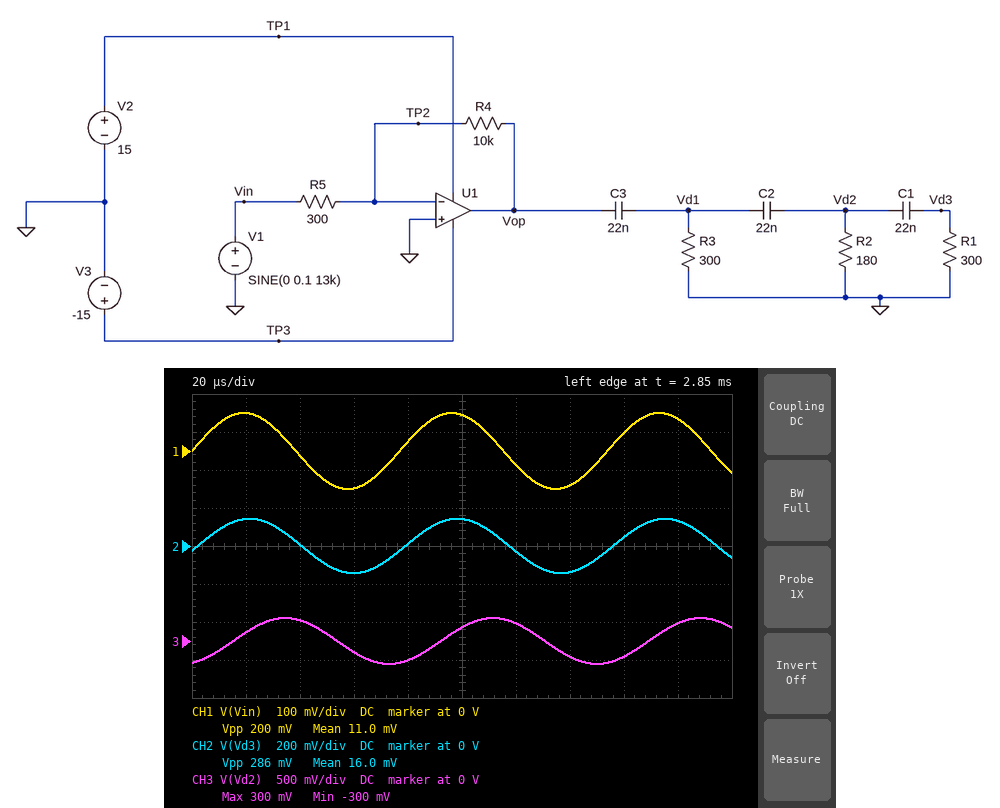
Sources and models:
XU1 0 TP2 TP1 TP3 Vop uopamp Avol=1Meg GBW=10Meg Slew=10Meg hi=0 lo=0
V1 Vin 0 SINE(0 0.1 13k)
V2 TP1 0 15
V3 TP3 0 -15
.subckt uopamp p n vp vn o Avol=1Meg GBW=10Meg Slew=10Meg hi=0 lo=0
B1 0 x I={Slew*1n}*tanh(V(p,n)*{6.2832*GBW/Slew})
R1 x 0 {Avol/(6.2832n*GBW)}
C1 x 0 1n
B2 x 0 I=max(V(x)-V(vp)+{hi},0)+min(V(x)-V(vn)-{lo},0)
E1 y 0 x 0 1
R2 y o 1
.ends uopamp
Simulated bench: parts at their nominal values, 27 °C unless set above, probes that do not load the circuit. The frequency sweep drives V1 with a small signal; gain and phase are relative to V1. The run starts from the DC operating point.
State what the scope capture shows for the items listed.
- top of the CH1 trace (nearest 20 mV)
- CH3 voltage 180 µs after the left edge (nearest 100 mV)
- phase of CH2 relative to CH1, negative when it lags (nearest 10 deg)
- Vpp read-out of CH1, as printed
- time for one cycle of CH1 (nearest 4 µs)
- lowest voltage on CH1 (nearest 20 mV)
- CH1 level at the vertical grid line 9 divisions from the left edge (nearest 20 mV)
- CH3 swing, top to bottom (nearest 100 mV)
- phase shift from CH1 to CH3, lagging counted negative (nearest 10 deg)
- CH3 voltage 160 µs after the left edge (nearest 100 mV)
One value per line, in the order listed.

100 mV
200 mV
-10 deg
200 mV
76 µs
-100 mV
80 mV
600 mV
-70 deg
-200 mV
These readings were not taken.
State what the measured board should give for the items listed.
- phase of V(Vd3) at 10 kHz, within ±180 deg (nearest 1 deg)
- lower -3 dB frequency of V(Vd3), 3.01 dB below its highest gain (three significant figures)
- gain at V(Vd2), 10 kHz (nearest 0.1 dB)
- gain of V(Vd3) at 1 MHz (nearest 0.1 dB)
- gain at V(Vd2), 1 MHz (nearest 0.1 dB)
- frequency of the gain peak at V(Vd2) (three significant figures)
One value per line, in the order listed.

6 deg
85.9 kHz
6.7 dB
19.2 dB
19.2 dB
207 kHz
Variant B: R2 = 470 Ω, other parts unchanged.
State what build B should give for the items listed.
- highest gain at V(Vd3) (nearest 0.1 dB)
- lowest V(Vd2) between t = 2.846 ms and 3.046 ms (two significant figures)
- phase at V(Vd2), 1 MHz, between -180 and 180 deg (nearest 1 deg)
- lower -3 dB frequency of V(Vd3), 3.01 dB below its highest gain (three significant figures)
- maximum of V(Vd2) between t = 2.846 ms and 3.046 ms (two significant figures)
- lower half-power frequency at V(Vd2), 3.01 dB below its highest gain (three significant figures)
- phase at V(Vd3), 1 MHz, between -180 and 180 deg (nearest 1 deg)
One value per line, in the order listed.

27.7 dB
-510 mV
112 deg
69.0 kHz
510 mV
63.8 kHz
113 deg
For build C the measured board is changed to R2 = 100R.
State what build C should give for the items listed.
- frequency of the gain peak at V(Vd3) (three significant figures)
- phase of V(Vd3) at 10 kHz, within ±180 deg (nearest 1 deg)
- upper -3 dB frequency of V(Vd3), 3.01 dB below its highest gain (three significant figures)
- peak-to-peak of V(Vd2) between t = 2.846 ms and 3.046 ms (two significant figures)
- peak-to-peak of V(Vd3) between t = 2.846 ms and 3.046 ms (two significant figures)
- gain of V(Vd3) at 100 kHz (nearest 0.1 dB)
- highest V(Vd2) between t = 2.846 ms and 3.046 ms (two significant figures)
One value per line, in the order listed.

248 kHz
14 deg
599 kHz
380 mV
180 mV
22.4 dB
190 mV
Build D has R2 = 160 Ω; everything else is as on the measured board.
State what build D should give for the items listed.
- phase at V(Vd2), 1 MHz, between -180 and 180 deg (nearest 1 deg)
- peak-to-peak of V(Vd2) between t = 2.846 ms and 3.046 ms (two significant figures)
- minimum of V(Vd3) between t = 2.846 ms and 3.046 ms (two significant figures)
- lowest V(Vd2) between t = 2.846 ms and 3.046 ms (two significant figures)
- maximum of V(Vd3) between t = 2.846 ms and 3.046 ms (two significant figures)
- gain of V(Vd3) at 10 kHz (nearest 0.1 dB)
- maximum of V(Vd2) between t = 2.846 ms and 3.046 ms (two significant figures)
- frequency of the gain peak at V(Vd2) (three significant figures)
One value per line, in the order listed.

115 deg
550 mV
-130 mV
-280 mV
130 mV
-2.4 dB
280 mV
214 kHz
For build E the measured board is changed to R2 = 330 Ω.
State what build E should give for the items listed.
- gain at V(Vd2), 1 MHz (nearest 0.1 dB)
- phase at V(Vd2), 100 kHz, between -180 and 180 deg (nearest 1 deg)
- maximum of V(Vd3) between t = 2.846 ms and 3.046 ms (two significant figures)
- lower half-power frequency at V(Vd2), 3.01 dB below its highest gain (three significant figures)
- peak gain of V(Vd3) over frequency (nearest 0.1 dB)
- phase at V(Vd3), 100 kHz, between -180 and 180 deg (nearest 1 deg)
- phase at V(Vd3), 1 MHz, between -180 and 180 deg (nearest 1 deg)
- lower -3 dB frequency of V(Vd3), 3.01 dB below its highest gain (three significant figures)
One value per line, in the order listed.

19.3 dB
-150 deg
210 mV
68.9 kHz
27.5 dB
-137 deg
114 deg
73.7 kHz
